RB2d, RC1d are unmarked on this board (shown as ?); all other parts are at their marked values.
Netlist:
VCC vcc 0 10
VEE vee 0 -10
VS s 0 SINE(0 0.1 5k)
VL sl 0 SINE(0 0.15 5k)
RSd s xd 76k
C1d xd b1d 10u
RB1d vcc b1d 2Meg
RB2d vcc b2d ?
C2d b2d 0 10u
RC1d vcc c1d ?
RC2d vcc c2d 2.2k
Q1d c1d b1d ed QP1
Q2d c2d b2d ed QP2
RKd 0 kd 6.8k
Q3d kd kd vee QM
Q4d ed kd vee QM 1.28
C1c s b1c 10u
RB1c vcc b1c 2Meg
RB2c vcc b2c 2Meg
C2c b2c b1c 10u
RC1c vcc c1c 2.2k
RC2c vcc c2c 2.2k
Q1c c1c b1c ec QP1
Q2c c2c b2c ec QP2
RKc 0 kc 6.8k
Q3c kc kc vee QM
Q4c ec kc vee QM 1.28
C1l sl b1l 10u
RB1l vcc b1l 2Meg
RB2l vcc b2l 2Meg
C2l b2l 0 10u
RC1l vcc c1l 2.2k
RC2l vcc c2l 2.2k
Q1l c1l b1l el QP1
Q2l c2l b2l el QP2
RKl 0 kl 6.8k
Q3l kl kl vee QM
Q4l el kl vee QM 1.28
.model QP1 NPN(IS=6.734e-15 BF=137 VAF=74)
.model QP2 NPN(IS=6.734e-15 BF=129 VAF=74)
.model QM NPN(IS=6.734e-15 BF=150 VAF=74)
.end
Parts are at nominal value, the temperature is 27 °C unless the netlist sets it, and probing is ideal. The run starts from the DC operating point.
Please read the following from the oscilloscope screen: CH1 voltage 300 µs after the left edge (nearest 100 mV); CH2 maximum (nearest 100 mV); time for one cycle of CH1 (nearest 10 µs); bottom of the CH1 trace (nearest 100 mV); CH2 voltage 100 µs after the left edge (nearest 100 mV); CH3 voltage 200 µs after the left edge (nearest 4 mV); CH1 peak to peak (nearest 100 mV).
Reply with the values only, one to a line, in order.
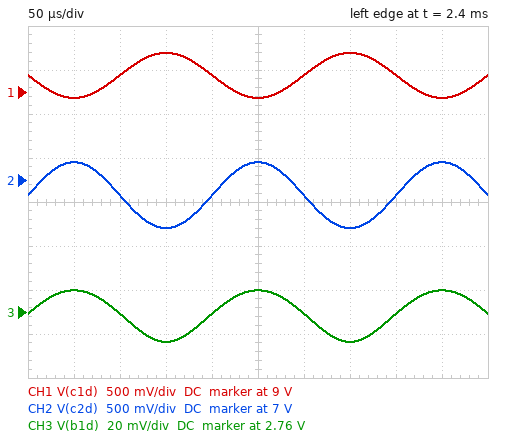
9.2 V
7.2 V
200 µs
8.9 V
6.8 V
2.760 V
500 mV
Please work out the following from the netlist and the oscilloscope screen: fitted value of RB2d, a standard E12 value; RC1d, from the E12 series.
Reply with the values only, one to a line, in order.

680 kΩ
1.5 kΩ
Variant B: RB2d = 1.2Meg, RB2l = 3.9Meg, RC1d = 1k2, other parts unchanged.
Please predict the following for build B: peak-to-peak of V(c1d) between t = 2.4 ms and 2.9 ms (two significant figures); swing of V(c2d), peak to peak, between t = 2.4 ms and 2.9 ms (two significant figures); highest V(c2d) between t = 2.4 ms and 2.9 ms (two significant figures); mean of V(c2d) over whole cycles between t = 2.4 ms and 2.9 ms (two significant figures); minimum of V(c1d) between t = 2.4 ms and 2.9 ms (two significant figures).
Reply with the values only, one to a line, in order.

430 mV
780 mV
7.8 V
7.4 V
8.9 V
